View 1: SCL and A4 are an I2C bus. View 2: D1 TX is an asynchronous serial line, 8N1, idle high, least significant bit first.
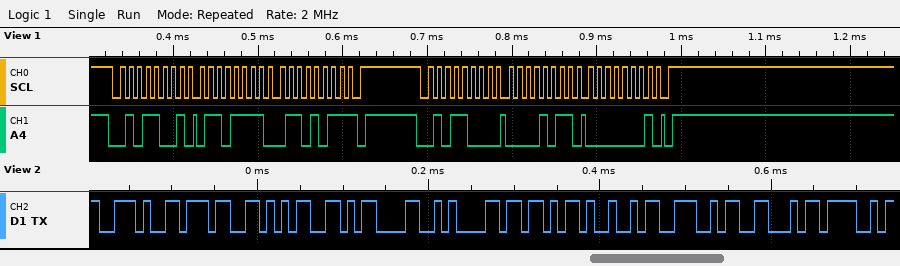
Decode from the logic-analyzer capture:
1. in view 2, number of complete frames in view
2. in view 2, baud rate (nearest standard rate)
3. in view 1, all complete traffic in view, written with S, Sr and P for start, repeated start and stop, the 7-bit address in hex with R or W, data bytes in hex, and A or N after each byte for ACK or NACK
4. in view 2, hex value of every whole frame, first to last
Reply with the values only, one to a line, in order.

10
115200 baud
S 2CR A 6F A 6B N P S 2CW A 0B A 01 A P
2E 37 35 0D 0A 5B 49 4E 46 4F
